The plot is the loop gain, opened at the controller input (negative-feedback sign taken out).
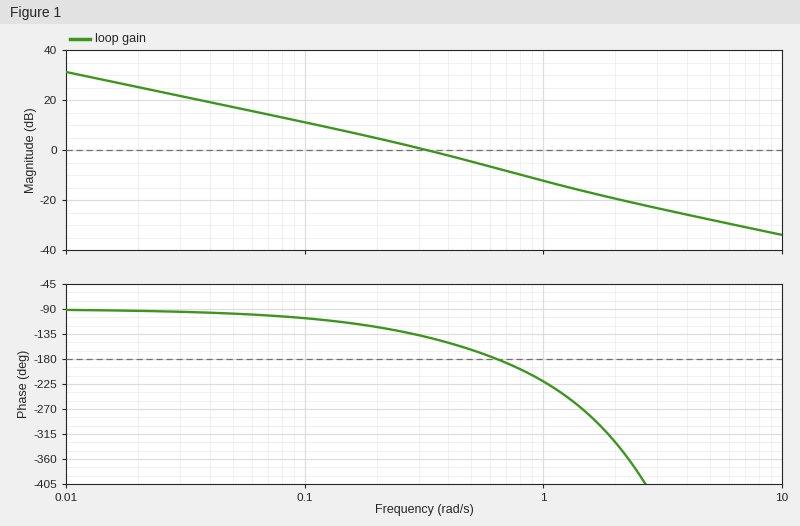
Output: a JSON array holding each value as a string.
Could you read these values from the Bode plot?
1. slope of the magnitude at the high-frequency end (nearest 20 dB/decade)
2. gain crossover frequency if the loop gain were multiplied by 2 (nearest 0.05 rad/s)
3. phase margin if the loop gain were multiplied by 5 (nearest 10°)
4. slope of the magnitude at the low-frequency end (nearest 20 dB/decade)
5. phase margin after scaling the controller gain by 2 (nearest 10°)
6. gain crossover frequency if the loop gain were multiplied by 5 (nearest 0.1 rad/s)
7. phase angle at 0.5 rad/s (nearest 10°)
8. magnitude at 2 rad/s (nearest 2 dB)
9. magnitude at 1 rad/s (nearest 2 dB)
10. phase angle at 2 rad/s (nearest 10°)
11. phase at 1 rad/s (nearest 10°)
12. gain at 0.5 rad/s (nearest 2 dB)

["-20 dB/decade", "0.55 rad/s", "-60°", "-20 dB/decade", "10°", "1.2 rad/s", "-160°", "-20 dB", "-12 dB", "-330°", "-220°", "-4 dB"]
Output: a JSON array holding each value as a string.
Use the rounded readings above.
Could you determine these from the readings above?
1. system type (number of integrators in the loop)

["1"]
